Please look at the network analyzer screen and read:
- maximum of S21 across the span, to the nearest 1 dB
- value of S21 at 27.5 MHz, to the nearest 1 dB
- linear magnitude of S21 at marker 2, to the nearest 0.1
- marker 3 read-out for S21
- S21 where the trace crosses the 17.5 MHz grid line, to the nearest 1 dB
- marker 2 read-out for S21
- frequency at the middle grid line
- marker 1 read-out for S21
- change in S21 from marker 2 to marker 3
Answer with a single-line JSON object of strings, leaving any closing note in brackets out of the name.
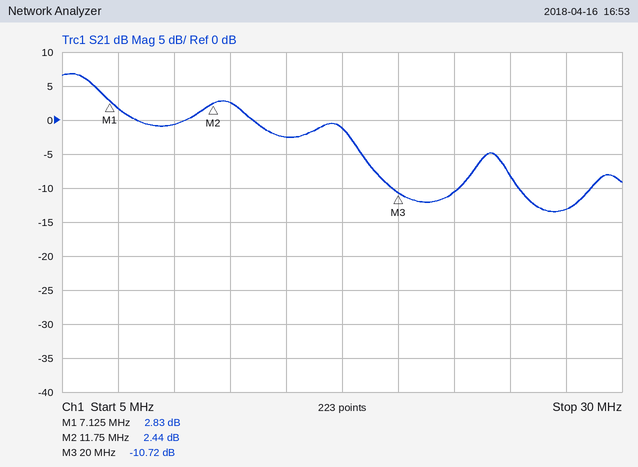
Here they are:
{"maximum of S21 across the span, to the nearest 1 dB": "7 dB", "value of S21 at 27.5 MHz, to the nearest 1 dB": "-13 dB", "linear magnitude of S21 at marker 2, to the nearest 0.1": "1.3", "marker 3 read-out for S21": "-10.72 dB", "S21 where the trace crosses the 17.5 MHz grid line, to the nearest 1 dB": "-1 dB", "marker 2 read-out for S21": "2.44 dB", "frequency at the middle grid line": "17.5 MHz", "marker 1 read-out for S21": "2.83 dB", "change in S21 from marker 2 to marker 3": "-13.16 dB"}
